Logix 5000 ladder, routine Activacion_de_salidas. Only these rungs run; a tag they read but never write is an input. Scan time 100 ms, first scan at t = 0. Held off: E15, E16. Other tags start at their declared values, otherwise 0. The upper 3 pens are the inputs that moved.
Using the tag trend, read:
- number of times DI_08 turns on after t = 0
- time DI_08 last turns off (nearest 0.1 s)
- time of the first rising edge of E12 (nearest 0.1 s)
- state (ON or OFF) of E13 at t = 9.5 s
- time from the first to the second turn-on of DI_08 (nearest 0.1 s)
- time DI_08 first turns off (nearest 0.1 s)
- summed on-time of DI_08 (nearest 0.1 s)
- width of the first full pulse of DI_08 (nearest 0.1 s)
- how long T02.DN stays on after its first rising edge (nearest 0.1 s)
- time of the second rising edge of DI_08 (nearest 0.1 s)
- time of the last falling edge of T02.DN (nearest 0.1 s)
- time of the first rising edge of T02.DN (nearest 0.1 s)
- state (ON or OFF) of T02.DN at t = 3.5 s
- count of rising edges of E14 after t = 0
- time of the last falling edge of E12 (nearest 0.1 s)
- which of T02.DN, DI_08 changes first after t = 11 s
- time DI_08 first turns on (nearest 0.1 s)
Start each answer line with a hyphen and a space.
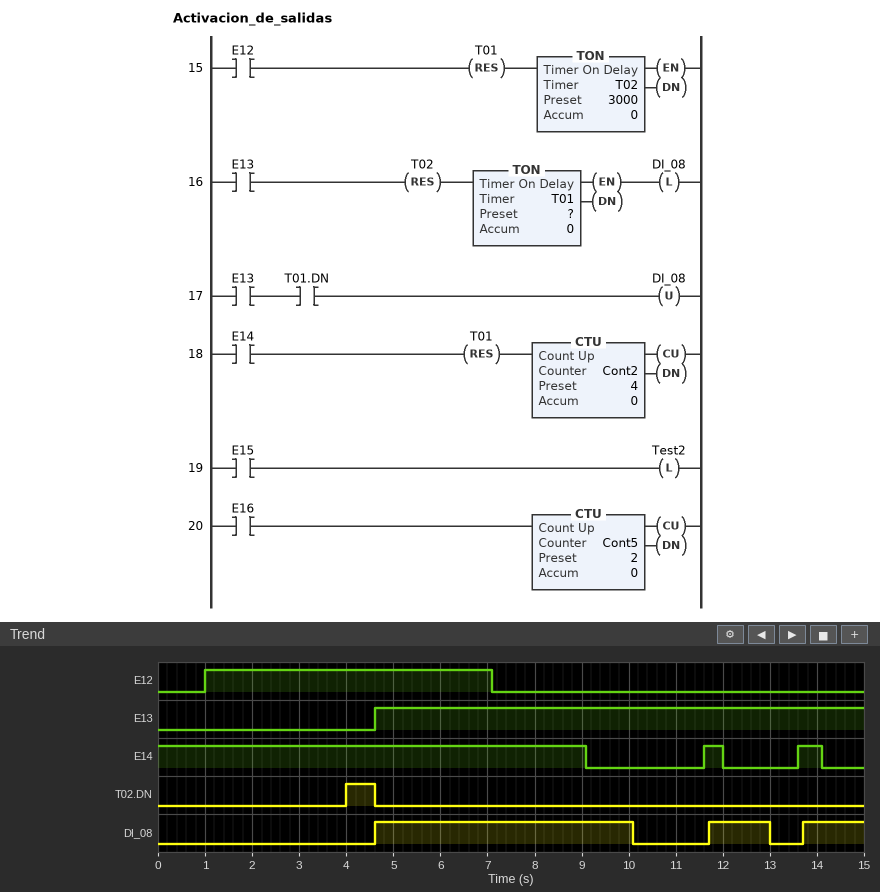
- 3
- 13.0 s
- 1.0 s
- ON
- 7.1 s
- 10.1 s
- 8.1 s
- 5.5 s
- 0.6 s
- 11.7 s
- 4.6 s
- 4.0 s
- OFF
- 2
- 7.1 s
- DI_08
- 4.6 s
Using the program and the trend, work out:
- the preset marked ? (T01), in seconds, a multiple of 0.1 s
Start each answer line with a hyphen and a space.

- 1.0 s
